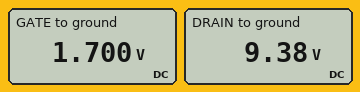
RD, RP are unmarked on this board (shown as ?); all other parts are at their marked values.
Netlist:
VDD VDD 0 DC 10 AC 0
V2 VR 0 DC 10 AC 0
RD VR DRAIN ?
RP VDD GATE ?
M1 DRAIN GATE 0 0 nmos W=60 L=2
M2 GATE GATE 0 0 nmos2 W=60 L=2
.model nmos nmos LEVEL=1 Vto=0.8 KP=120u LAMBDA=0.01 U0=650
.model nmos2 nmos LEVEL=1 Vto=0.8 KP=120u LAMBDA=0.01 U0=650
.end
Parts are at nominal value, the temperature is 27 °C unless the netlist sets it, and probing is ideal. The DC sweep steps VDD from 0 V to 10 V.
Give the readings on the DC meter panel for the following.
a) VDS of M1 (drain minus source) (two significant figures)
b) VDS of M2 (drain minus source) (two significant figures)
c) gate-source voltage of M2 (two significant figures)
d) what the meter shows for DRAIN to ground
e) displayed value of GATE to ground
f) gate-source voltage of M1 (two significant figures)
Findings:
9.4 V
1.7 V
1.7 V
9.38 V
1.700 V
1.7 V
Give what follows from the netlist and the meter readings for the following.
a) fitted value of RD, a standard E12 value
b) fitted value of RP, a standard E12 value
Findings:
390 Ω
5.6 kΩ
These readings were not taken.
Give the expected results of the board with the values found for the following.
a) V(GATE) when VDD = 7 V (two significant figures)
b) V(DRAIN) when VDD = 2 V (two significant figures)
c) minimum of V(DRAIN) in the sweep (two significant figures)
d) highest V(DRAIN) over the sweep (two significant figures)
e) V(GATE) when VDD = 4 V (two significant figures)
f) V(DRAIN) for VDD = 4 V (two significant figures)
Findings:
1.5 V
9.9 V
9.4 V
10 V
1.3 V
9.8 V
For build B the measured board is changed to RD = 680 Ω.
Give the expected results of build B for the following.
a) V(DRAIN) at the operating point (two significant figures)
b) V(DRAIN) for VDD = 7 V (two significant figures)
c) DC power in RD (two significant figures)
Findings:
8.9 V
9.3 V
1.7 mW
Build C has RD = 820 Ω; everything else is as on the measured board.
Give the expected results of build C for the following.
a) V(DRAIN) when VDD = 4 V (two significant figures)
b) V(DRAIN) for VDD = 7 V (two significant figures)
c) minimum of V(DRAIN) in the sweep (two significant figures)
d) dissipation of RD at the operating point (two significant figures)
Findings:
9.6 V
9.1 V
8.7 V
2.1 mW
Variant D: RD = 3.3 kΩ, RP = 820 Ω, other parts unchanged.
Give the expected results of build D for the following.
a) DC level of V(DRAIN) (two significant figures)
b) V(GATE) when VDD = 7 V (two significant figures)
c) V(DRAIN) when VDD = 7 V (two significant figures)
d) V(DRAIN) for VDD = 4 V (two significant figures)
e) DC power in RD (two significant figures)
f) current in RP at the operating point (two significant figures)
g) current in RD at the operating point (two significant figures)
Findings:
410 mV
2.5 V
550 mV
1.8 V
28 mW
8.6 mA
2.9 mA
